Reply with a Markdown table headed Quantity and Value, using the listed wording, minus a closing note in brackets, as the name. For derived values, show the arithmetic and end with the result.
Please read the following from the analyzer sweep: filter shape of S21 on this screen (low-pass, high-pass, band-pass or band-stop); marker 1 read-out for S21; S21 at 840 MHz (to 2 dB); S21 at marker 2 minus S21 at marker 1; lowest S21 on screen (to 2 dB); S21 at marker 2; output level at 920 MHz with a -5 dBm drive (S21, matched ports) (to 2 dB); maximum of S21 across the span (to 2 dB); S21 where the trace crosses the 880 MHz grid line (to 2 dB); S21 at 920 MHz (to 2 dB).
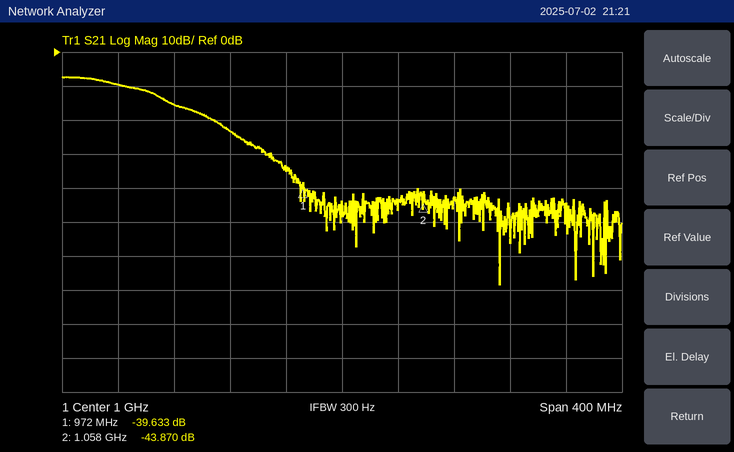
| Quantity | Value |
|---|---|
| filter shape of S21 on this screen | low-pass |
| marker 1 read-out for S21 | -39.633 dB |
| S21 at 840 MHz | -10 dB |
| S21 at marker 2 minus S21 at marker 1 | -43.87 − (-39.633) = -4.237 dB |
| lowest S21 on screen | -68 dB |
| S21 at marker 2 | -43.870 dB |
| output level at 920 MHz with a -5 dBm drive (S21, matched ports) | -5 dBm + (-24 dB) = -28 dBm |
| maximum of S21 across the span | -8 dB |
| S21 where the trace crosses the 880 MHz grid line | -16 dB |
| S21 at 920 MHz | -24 dB |
